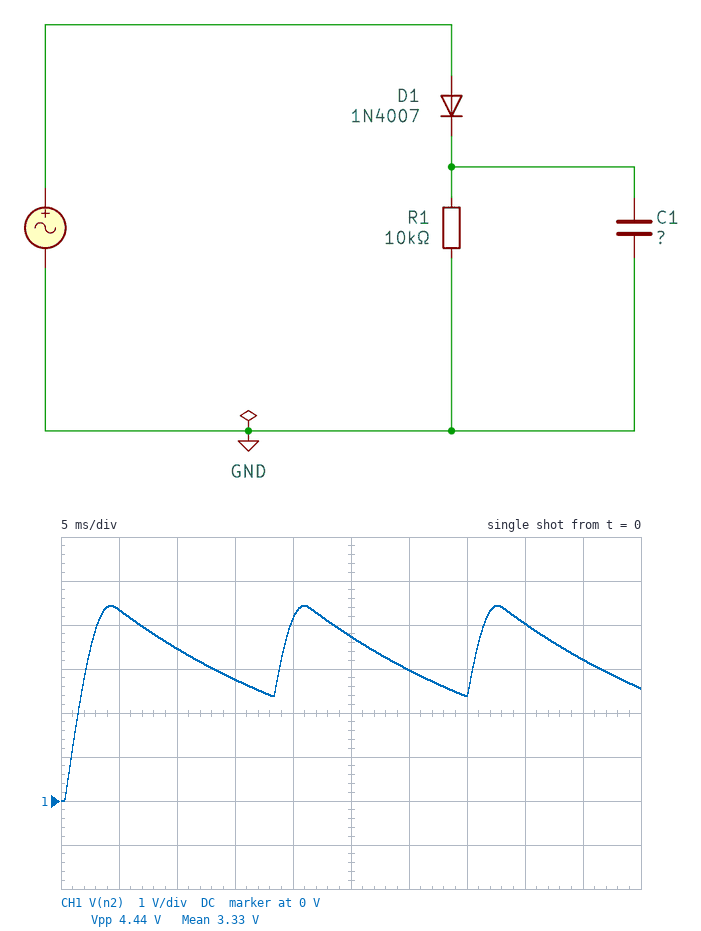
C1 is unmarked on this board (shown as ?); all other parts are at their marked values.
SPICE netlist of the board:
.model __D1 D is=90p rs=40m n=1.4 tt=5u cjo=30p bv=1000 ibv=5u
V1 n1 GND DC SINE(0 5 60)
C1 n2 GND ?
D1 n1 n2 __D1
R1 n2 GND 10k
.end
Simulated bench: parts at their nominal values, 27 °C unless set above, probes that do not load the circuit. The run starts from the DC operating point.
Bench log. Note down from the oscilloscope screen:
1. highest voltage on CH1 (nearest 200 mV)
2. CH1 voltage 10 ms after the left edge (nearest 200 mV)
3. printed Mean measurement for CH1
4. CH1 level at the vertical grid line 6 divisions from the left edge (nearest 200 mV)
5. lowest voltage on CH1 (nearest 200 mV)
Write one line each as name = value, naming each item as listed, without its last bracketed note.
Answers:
highest voltage on CH1 = 4.4 V
CH1 voltage 10 ms after the left edge = 3.4 V
printed Mean measurement for CH1 = 3.33 V
CH1 level at the vertical grid line 6 divisions from the left edge = 3.0 V
lowest voltage on CH1 = 0 V
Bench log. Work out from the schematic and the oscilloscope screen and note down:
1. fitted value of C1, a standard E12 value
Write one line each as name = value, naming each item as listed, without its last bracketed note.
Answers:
fitted value of C1, a standard E12 value = 2.2 µF
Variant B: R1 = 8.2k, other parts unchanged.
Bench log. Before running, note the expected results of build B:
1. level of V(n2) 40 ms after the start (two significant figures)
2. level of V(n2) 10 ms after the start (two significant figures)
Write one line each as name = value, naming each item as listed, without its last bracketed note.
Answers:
level of V(n2) 40 ms after the start = 3.9 V
level of V(n2) 10 ms after the start = 3.3 V
